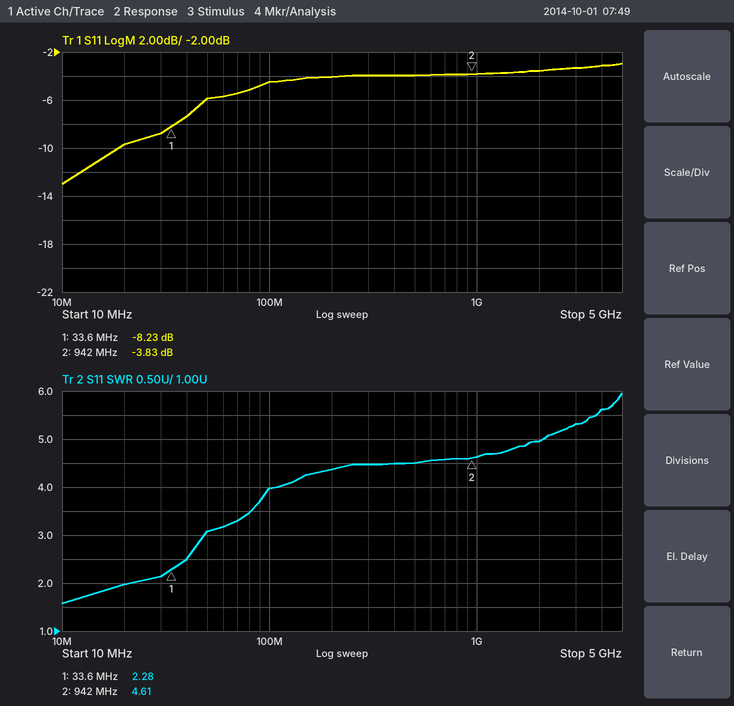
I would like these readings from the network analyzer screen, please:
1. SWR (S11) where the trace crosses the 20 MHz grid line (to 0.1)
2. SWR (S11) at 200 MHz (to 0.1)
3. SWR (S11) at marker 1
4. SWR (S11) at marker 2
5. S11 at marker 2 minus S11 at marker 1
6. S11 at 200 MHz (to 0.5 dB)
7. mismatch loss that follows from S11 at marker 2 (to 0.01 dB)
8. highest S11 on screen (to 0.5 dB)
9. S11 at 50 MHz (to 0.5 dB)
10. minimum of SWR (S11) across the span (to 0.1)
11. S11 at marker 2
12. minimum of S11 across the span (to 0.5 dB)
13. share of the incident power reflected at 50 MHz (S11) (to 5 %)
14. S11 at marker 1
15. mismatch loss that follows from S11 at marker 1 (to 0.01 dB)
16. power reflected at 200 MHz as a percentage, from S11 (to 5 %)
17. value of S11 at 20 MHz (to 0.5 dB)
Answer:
2.0
4.4
2.28
4.61
4.40 dB
-4.0 dB
2.32 dB
-3.0 dB
-6.0 dB
1.6
-3.83 dB
-13.0 dB
25 %
-8.23 dB
0.71 dB
40 %
-9.5 dB
